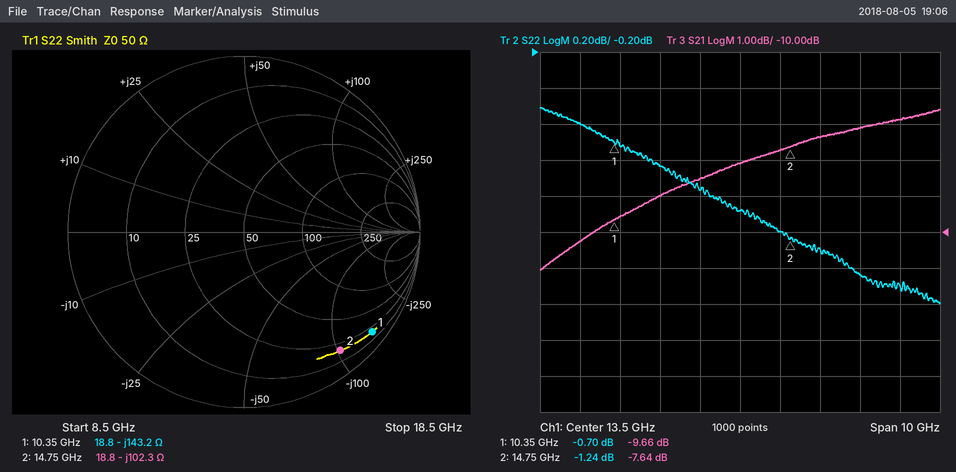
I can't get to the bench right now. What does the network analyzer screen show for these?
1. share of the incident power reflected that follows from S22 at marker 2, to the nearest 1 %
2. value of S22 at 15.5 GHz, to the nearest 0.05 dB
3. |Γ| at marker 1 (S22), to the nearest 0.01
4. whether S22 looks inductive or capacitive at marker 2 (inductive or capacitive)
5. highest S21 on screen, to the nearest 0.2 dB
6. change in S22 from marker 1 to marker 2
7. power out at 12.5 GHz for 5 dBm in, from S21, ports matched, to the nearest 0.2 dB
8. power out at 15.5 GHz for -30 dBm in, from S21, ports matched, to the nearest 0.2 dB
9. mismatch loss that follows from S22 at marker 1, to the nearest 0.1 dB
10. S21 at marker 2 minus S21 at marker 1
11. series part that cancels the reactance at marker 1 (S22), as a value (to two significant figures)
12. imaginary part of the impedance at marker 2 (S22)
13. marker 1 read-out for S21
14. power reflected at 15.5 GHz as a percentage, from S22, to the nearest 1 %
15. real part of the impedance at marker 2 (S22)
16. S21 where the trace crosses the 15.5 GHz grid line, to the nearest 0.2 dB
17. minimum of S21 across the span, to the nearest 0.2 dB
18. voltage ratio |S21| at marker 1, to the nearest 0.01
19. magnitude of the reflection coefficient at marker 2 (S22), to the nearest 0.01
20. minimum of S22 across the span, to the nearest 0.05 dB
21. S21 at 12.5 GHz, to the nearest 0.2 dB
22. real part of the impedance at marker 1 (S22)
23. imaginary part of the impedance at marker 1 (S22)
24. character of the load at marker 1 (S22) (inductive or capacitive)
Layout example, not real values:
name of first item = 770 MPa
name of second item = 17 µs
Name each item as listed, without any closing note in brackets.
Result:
share of the incident power reflected that follows from S22 at marker 2, to the nearest 1 % = 75 %
value of S22 at 15.5 GHz, to the nearest 0.05 dB = -1.30 dB
|Γ| at marker 1 (S22), to the nearest 0.01 = 0.92
whether S22 looks inductive or capacitive at marker 2 = capacitive
highest S21 on screen, to the nearest 0.2 dB = -6.6 dB
change in S22 from marker 1 to marker 2 = -0.54 dB
power out at 12.5 GHz for 5 dBm in, from S21, ports matched, to the nearest 0.2 dB = -3.6 dBm
power out at 15.5 GHz for -30 dBm in, from S21, ports matched, to the nearest 0.2 dB = -37.4 dBm
mismatch loss that follows from S22 at marker 1, to the nearest 0.1 dB = 8.3 dB
S21 at marker 2 minus S21 at marker 1 = 2.02 dB
series part that cancels the reactance at marker 1 (S22), as a value = 2.2 nH
imaginary part of the impedance at marker 2 = -102.3 Ω
marker 1 read-out for S21 = -9.66 dB
power reflected at 15.5 GHz as a percentage, from S22, to the nearest 1 % = 74 %
real part of the impedance at marker 2 = 18.8 Ω
S21 where the trace crosses the 15.5 GHz grid line, to the nearest 0.2 dB = -7.4 dB
minimum of S21 across the span, to the nearest 0.2 dB = -11.0 dB
voltage ratio |S21| at marker 1, to the nearest 0.01 = 0.33
magnitude of the reflection coefficient at marker 2 (S22), to the nearest 0.01 = 0.87
minimum of S22 across the span, to the nearest 0.05 dB = -1.60 dB
S21 at 12.5 GHz, to the nearest 0.2 dB = -8.6 dB
real part of the impedance at marker 1 = 18.8 Ω
imaginary part of the impedance at marker 1 = -143.2 Ω
character of the load at marker 1 (S22) = capacitive
